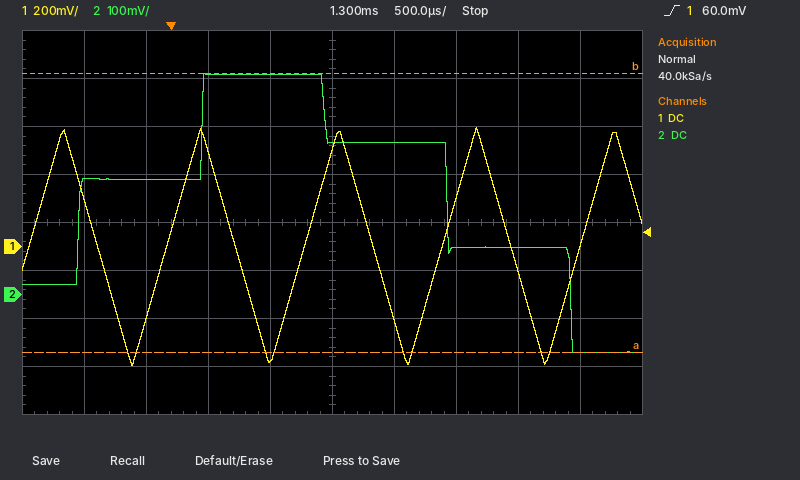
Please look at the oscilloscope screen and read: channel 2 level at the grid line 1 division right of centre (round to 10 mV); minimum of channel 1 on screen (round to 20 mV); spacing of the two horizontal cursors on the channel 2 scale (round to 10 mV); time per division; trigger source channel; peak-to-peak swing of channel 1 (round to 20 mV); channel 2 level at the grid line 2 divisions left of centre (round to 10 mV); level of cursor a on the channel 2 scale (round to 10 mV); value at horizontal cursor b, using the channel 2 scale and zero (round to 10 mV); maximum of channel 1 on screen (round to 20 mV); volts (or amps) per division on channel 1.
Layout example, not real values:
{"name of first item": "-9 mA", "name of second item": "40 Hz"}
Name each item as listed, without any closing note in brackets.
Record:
{"channel 2 level at the grid line 1 division right of centre": "320 mV", "minimum of channel 1 on screen": "-500 mV", "spacing of the two horizontal cursors on the channel 2 scale": "580 mV", "time per division": "500 µs", "trigger source channel": "channel 1", "peak-to-peak swing of channel 1": "1.00 V", "channel 2 level at the grid line 2 divisions left of centre": "460 mV", "level of cursor a on the channel 2 scale": "-120 mV", "value at horizontal cursor b, using the channel 2 scale and zero": "460 mV", "maximum of channel 1 on screen": "500 mV", "volts (or amps) per division on channel 1": "200 mV"}
